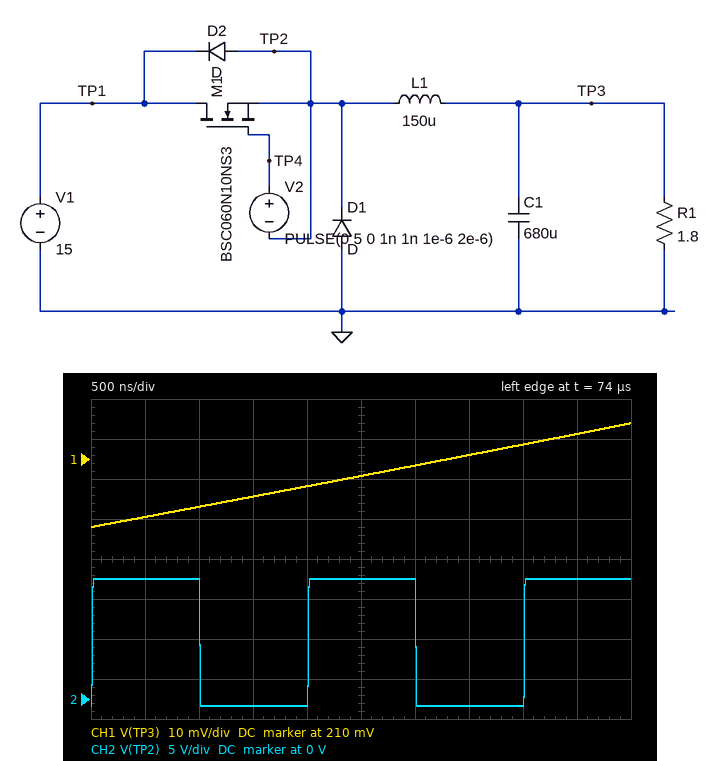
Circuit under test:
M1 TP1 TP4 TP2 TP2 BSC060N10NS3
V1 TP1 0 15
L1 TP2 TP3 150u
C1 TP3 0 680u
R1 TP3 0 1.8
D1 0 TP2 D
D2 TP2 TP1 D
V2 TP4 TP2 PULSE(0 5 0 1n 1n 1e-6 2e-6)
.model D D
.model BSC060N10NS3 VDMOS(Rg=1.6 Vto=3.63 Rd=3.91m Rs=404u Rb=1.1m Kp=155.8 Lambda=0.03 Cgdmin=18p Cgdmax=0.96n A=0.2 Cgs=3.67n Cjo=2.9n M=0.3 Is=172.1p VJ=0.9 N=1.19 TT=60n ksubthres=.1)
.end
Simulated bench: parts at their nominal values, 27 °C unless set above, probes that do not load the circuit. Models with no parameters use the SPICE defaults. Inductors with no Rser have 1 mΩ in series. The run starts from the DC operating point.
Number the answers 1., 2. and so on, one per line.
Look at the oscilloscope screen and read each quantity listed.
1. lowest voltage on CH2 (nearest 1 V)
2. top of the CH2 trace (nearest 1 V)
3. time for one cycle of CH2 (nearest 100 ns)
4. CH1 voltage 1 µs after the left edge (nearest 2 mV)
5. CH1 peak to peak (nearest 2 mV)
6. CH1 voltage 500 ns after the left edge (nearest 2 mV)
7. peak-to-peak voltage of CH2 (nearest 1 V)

1. -1 V
2. 15 V
3. 2.0 µs
4. 198 mV
5. 26 mV
6. 196 mV
7. 16 V
